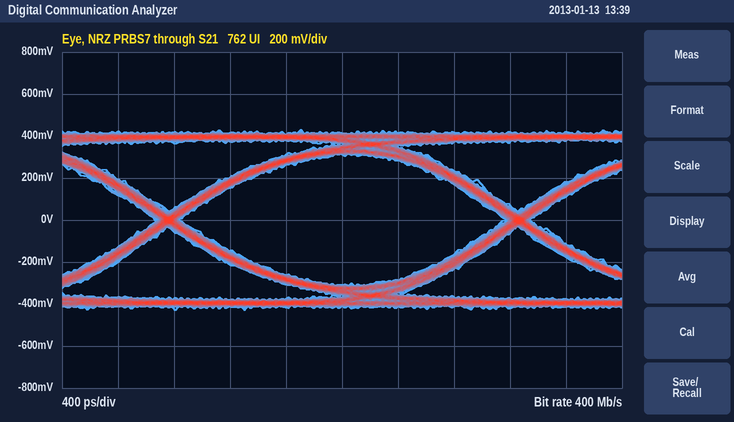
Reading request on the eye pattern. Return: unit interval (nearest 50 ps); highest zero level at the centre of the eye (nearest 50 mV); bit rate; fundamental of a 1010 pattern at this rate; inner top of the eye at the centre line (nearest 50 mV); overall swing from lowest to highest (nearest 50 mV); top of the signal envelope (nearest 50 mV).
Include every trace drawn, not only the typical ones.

2.50 ns
-300 mV
400 Mb/s
200 MHz
300 mV
850 mV
450 mV
